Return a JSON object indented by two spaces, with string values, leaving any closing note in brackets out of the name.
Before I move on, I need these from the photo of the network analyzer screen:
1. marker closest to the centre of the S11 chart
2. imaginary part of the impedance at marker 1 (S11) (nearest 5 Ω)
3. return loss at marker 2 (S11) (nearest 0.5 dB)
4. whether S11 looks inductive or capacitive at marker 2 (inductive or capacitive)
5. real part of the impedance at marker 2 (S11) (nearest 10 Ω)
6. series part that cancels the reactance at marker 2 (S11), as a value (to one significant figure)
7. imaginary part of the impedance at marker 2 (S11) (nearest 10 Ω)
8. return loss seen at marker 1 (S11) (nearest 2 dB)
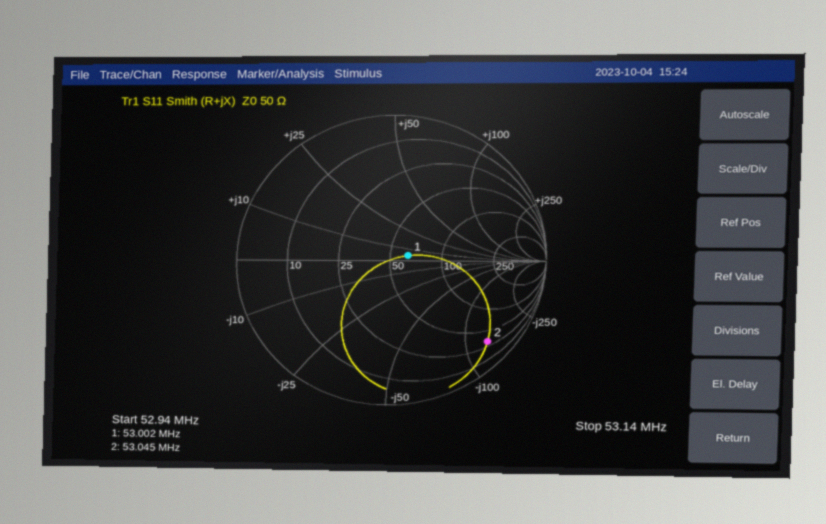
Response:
{
  "marker closest to the centre of the S11 chart": "marker 1",
  "imaginary part of the impedance at marker 1 (S11)": "+5 Ω",
  "return loss at marker 2 (S11)": "1.5 dB",
  "whether S11 looks inductive or capacitive at marker 2": "capacitive",
  "real part of the impedance at marker 2 (S11)": "30 Ω",
  "series part that cancels the reactance at marker 2 (S11), as a value": "400 nH",
  "imaginary part of the impedance at marker 2 (S11)": "-130 Ω",
  "return loss seen at marker 1 (S11)": "18 dB"
}
